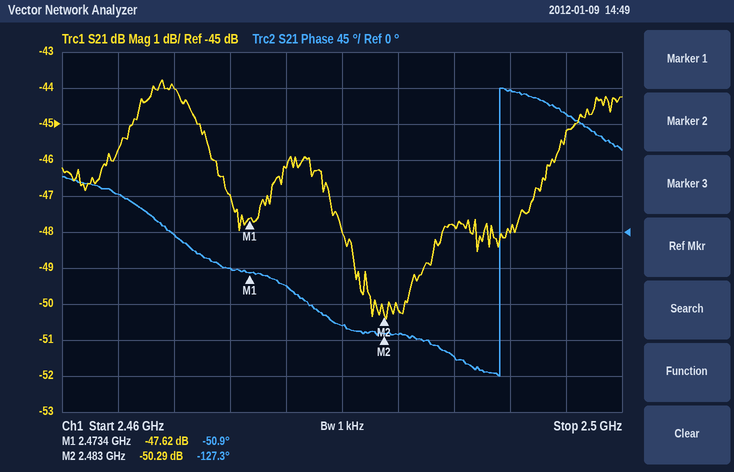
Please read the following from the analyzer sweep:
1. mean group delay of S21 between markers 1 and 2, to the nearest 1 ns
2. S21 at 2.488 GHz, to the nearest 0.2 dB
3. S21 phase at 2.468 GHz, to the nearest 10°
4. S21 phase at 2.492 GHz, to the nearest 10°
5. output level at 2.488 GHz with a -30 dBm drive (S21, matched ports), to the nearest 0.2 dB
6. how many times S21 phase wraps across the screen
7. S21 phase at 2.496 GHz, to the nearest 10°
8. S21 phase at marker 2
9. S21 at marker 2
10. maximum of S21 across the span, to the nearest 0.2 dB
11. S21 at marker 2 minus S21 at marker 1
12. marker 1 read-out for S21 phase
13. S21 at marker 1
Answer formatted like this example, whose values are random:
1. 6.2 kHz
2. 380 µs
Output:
1. 22 ns
2. -47.8 dB
3. 0°
4. 180°
5. -77.8 dBm
6. 1
7. 150°
8. -127.3°
9. -50.29 dB
10. -43.8 dB
11. -2.67 dB
12. -50.9°
13. -47.62 dB
